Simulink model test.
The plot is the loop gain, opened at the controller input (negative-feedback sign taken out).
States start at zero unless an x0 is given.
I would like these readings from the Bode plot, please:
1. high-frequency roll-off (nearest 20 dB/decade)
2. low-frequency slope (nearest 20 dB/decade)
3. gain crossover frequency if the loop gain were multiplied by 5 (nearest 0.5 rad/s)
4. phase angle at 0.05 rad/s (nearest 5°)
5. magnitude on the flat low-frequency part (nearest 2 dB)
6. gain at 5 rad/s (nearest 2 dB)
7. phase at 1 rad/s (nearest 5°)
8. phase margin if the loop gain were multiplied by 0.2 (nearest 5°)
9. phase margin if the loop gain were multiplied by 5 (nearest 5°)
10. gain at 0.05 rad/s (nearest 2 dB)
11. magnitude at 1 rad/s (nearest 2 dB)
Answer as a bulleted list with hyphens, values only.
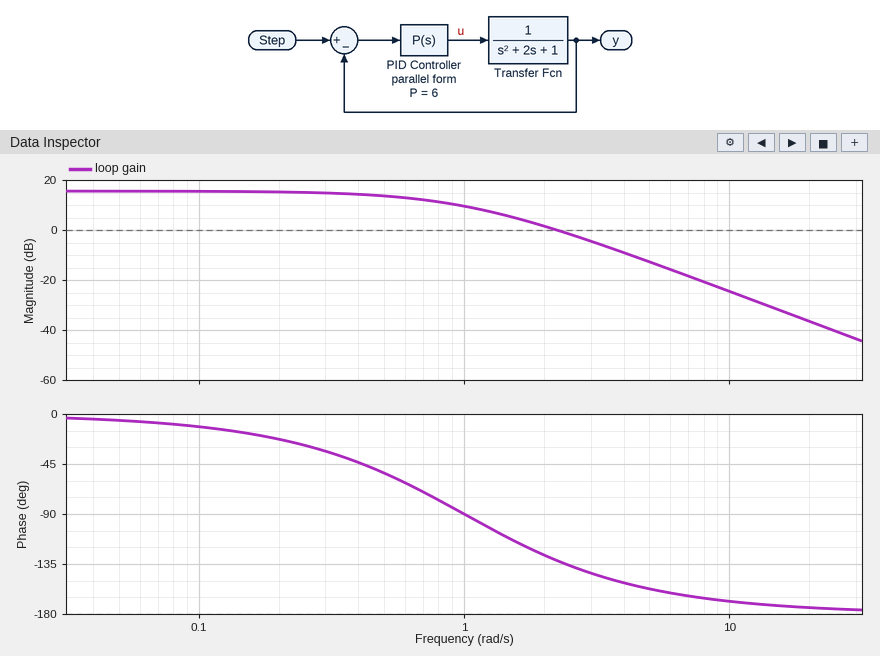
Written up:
- -40 dB/decade
- 0 dB/decade
- 5.5 rad/s
- -5°
- 16 dB
- -12 dB
- -90°
- 130°
- 20°
- 16 dB
- 10 dB
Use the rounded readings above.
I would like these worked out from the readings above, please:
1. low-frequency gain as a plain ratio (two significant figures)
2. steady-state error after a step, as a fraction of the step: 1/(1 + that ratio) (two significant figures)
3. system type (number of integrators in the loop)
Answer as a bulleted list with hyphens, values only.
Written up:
- 6.3
- 0.14
- 0
